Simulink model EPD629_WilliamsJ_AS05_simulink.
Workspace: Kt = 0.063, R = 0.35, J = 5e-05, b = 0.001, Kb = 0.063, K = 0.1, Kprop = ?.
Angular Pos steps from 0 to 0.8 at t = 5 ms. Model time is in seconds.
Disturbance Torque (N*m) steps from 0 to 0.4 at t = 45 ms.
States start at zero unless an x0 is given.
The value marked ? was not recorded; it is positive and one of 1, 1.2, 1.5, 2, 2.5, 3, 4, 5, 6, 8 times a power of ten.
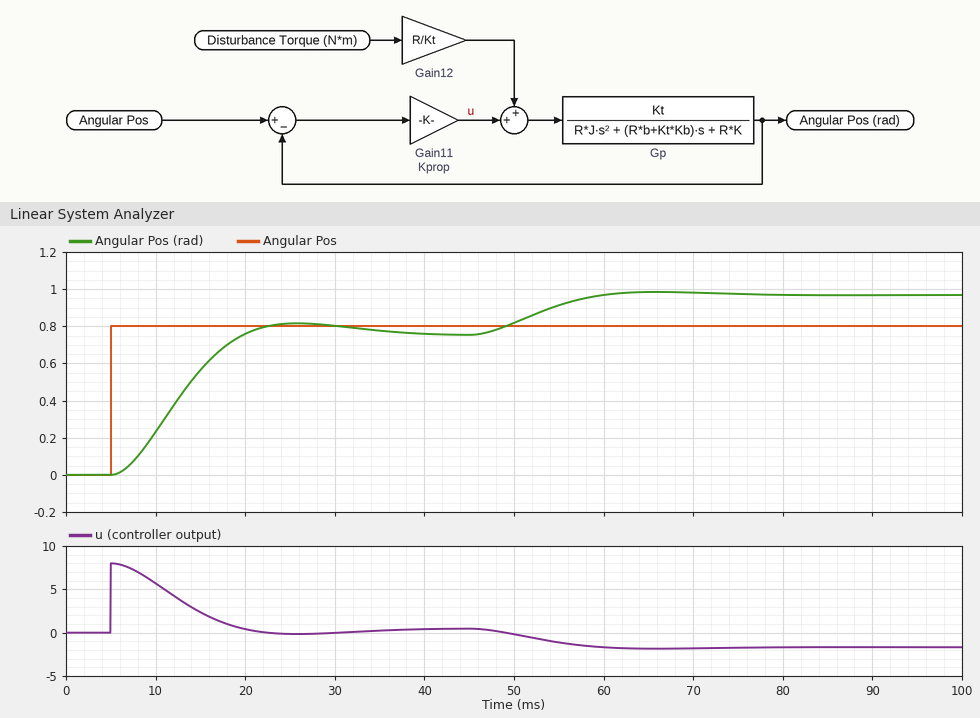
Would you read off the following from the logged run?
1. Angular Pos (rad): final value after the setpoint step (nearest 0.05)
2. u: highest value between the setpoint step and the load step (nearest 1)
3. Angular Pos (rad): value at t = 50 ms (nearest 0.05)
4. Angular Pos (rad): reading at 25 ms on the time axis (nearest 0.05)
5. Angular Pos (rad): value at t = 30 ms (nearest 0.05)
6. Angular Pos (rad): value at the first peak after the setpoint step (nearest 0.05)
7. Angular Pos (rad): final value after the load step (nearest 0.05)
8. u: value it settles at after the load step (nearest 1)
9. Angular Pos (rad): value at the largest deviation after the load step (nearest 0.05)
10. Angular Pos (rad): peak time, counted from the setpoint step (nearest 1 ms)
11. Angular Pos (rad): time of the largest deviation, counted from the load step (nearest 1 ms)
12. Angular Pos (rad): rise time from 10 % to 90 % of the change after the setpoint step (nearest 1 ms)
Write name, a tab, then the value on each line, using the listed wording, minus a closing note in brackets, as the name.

Angular Pos (rad): final value after the setpoint step	0.75
u: highest value between the setpoint step and the load step	8
Angular Pos (rad): value at t = 50 ms	0.80
Angular Pos (rad): reading at 25 ms on the time axis	0.80
Angular Pos (rad): value at t = 30 ms	0.80
Angular Pos (rad): value at the first peak after the setpoint step	0.80
Angular Pos (rad): final value after the load step	0.95
u: value it settles at after the load step	-2
Angular Pos (rad): value at the largest deviation after the load step	1.00
Angular Pos (rad): peak time, counted from the setpoint step	21 ms
Angular Pos (rad): time of the largest deviation, counted from the load step	21 ms
Angular Pos (rad): rise time from 10 % to 90 % of the change after the setpoint step	10 ms
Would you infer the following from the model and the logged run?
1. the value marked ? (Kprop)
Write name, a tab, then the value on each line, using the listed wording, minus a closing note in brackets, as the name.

the value marked ?	10
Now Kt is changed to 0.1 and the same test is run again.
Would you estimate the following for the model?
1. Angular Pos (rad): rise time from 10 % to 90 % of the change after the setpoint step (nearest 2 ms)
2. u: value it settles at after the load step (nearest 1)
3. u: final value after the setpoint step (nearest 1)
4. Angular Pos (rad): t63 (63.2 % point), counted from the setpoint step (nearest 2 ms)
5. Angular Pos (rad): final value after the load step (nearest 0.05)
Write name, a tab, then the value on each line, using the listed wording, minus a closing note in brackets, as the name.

Angular Pos (rad): rise time from 10 % to 90 % of the change after the setpoint step	10 ms
u: value it settles at after the load step	-1
u: final value after the setpoint step	0
Angular Pos (rad): t63 (63.2 % point), counted from the setpoint step	8 ms
Angular Pos (rad): final value after the load step	0.90
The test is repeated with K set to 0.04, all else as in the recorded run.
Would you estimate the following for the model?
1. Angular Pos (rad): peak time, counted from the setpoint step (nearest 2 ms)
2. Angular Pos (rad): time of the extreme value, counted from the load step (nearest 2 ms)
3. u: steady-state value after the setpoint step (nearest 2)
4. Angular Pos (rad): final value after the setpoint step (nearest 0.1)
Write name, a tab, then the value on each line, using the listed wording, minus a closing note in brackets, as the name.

Angular Pos (rad): peak time, counted from the setpoint step	22 ms
Angular Pos (rad): time of the extreme value, counted from the load step	22 ms
u: steady-state value after the setpoint step	0
Angular Pos (rad): final value after the setpoint step	0.8
